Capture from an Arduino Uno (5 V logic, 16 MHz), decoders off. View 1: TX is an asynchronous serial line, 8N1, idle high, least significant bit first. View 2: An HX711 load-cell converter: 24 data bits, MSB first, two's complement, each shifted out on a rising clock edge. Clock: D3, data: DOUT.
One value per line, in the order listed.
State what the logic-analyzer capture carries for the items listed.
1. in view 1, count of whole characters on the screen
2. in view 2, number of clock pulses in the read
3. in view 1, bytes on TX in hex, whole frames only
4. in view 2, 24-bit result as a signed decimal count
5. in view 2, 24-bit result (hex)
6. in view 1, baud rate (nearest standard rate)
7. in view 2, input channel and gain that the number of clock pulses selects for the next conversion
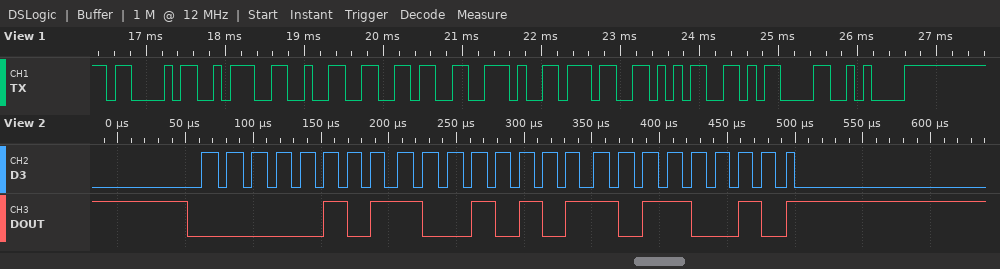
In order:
9
25
43 3A 32 36 2E 37 35 0D 0A
366002
0x0595B2
9600 baud
channel A, gain 128
